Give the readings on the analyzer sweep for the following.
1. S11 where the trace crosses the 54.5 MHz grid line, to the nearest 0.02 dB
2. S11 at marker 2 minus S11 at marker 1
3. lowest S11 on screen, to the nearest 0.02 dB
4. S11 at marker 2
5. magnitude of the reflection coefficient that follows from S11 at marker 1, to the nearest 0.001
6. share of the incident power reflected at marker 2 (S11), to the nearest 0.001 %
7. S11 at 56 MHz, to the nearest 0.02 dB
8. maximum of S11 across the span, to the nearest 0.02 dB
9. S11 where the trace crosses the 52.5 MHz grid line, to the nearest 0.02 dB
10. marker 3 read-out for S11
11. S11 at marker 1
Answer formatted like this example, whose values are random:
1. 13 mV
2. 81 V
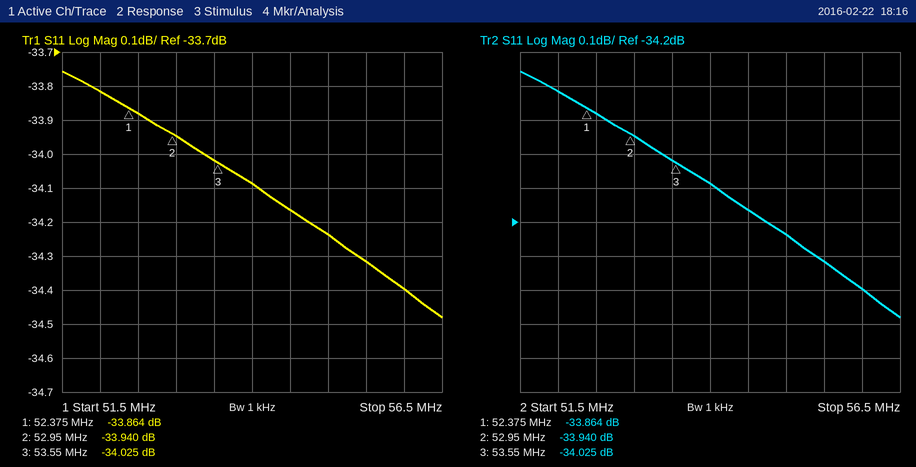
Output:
1. -34.16 dB
2. -0.076 dB
3. -34.48 dB
4. -33.940 dB
5. 0.020
6. 0.040 %
7. -34.40 dB
8. -33.76 dB
9. -33.88 dB
10. -34.025 dB
11. -33.864 dB
